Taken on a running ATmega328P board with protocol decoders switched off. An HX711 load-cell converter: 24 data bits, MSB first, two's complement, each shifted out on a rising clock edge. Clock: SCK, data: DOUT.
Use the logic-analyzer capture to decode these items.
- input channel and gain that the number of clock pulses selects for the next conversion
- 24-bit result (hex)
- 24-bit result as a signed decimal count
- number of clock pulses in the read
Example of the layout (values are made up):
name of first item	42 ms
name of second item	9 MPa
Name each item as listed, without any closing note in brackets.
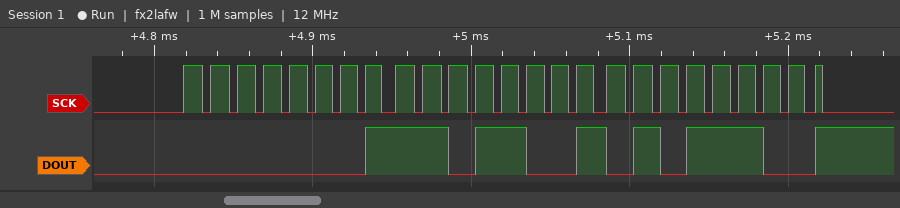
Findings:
input channel and gain that the number of clock pulses selects for the next conversion	channel A, gain 128
24-bit result	0x01D95C
24-bit result as a signed decimal count	121180
number of clock pulses in the read	25
